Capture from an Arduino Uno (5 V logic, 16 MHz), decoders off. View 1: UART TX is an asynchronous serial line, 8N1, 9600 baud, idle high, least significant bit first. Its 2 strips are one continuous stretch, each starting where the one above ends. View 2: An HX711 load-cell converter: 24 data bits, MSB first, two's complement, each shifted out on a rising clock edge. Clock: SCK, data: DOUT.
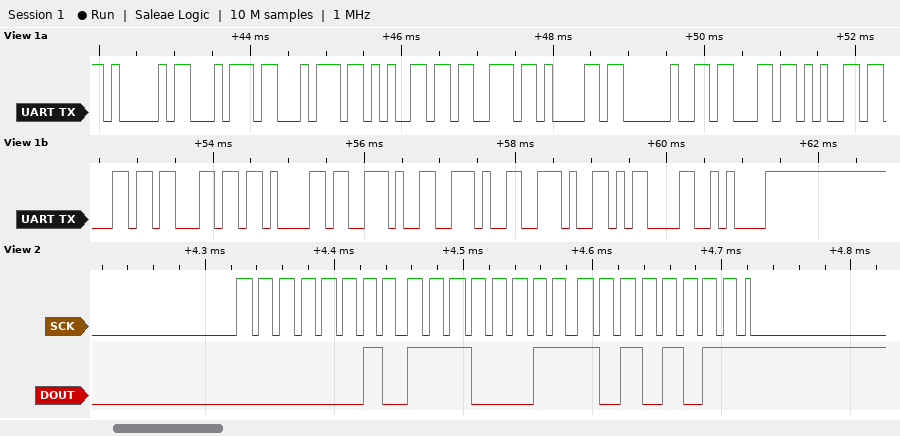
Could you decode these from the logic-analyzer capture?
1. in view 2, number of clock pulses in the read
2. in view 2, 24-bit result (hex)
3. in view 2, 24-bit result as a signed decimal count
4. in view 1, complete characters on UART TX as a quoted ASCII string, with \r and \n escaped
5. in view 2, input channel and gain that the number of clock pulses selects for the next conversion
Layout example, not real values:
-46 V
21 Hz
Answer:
25
0x02E3AB
189355
"Attesa cella...\r\n"
channel A, gain 128
